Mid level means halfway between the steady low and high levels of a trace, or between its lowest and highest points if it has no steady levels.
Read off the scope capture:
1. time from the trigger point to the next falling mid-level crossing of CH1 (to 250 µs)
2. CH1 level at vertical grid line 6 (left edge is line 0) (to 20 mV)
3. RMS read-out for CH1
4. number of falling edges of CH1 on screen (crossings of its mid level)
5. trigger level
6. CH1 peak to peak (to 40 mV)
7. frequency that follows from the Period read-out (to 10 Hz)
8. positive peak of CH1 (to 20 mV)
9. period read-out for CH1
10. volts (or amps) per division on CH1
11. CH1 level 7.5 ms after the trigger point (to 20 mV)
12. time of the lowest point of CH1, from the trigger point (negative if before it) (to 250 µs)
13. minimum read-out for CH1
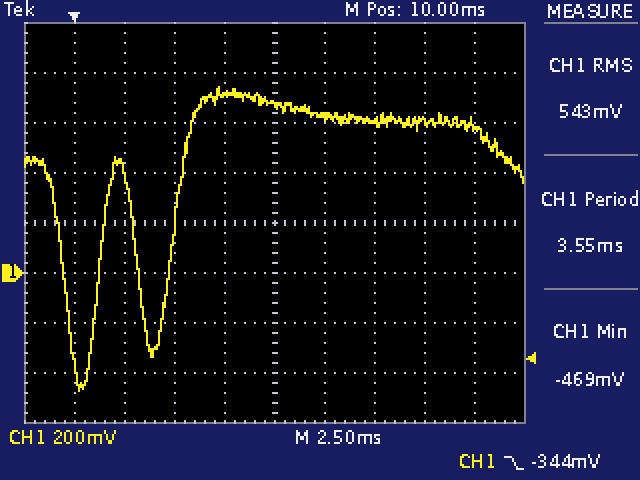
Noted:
3.00 ms
620 mV
543 mV
2
-344 mV
1.20 V
280 Hz
740 mV
3.55 ms
200 mV
720 mV
+250 µs
-469 mV
